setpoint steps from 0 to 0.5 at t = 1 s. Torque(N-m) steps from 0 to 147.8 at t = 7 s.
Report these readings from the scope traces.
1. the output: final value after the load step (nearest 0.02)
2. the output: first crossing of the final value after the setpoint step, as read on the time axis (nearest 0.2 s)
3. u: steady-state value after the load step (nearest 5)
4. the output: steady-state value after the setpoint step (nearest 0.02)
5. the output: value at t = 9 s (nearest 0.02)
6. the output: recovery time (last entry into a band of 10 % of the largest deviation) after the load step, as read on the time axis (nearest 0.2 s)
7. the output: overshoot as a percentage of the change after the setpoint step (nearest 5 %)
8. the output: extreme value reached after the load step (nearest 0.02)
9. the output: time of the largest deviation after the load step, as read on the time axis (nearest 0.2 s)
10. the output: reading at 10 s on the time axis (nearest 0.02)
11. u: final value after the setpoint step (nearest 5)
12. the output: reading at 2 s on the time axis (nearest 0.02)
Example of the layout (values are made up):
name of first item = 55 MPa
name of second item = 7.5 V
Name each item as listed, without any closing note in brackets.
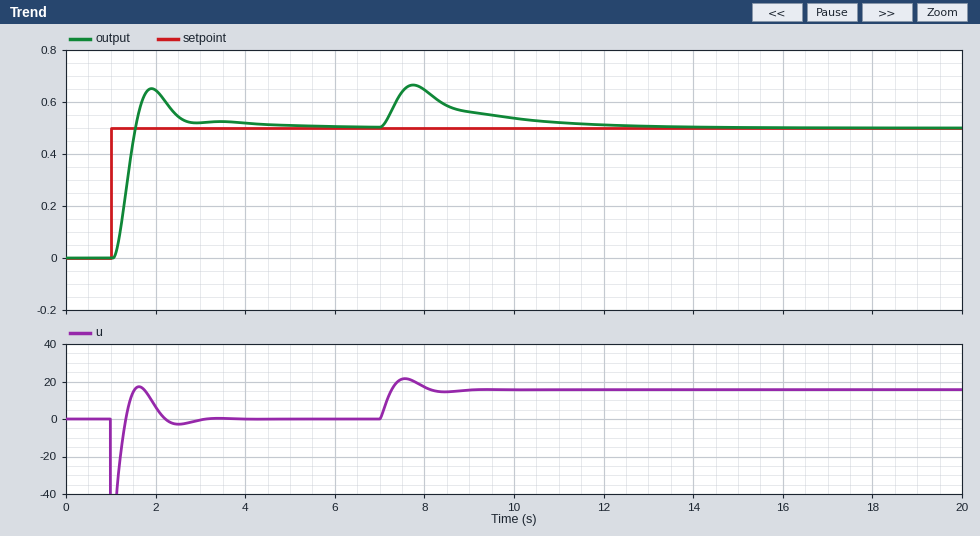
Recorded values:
the output: final value after the load step = 0.50
the output: first crossing of the final value after the setpoint step, as read on the time axis = 1.6 s
u: steady-state value after the load step = 15
the output: steady-state value after the setpoint step = 0.50
the output: value at t = 9 s = 0.56
the output: recovery time (last entry into a band of 10 % of the largest deviation) after the load step, as read on the time axis = 11.4 s
the output: overshoot as a percentage of the change after the setpoint step = 30 %
the output: extreme value reached after the load step = 0.66
the output: time of the largest deviation after the load step, as read on the time axis = 7.8 s
the output: reading at 10 s on the time axis = 0.54
u: final value after the setpoint step = 0
the output: reading at 2 s on the time axis = 0.64
